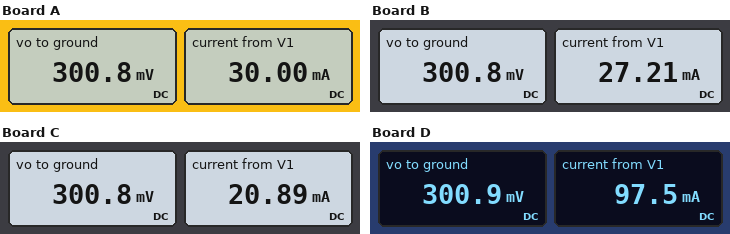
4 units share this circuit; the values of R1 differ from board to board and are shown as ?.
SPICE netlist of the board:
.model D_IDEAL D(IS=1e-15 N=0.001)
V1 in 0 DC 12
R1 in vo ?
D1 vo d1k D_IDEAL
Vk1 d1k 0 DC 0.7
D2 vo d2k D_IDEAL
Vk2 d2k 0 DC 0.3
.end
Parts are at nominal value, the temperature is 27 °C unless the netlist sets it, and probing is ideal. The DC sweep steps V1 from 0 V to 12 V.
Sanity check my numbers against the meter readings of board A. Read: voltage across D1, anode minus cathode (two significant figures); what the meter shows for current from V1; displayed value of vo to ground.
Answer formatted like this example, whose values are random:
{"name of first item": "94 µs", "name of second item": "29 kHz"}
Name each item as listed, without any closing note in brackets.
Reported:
{"voltage across D1, anode minus cathode": "-400 mV", "what the meter shows for current from V1": "30.00 mA", "displayed value of vo to ground": "300.8 mV"}
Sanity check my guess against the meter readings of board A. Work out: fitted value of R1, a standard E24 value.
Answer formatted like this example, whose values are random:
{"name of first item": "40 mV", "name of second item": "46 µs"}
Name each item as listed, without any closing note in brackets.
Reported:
{"fitted value of R1, a standard E24 value": "390 Ω"}
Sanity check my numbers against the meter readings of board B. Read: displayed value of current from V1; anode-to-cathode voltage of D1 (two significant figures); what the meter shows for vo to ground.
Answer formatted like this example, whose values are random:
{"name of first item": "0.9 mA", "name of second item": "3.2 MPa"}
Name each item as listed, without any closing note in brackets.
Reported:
{"displayed value of current from V1": "27.21 mA", "anode-to-cathode voltage of D1": "-400 mV", "what the meter shows for vo to ground": "300.8 mV"}
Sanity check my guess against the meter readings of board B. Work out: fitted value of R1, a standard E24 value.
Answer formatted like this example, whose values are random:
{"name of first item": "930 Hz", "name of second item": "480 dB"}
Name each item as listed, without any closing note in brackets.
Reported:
{"fitted value of R1, a standard E24 value": "430 Ω"}
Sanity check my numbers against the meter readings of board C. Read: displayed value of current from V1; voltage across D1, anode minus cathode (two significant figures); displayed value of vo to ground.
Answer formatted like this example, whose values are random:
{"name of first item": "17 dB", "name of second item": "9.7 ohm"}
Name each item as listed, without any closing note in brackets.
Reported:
{"displayed value of current from V1": "20.89 mA", "voltage across D1, anode minus cathode": "-400 mV", "displayed value of vo to ground": "300.8 mV"}
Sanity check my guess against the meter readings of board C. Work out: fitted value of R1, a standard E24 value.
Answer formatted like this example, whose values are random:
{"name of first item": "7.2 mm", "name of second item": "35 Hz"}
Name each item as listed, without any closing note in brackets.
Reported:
{"fitted value of R1, a standard E24 value": "560 Ω"}
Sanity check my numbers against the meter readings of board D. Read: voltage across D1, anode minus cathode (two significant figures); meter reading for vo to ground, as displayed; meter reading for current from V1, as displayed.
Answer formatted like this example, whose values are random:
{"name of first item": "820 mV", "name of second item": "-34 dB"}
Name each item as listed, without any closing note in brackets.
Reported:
{"voltage across D1, anode minus cathode": "-400 mV", "meter reading for vo to ground, as displayed": "300.9 mV", "meter reading for current from V1, as displayed": "97.5 mA"}
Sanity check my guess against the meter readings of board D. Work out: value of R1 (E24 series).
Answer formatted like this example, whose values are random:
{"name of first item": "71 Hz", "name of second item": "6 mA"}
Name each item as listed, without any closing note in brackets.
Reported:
{"value of R1": "120 Ω"}
